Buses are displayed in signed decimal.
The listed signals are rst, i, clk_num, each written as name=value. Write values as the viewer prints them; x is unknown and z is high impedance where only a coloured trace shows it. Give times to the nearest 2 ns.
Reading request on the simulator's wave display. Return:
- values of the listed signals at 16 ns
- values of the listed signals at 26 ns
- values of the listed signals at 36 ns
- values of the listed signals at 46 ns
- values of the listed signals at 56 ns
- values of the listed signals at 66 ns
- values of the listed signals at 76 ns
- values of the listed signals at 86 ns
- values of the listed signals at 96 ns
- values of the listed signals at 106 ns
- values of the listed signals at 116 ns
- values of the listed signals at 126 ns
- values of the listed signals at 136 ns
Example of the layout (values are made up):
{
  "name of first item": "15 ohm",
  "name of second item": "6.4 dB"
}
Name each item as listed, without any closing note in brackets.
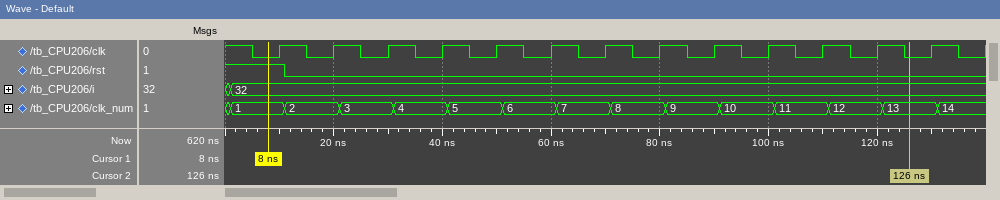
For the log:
{
  "values of the listed signals at 16 ns": "rst=0, i=32, clk_num=2",
  "values of the listed signals at 26 ns": "rst=0, i=32, clk_num=3",
  "values of the listed signals at 36 ns": "rst=0, i=32, clk_num=4",
  "values of the listed signals at 46 ns": "rst=0, i=32, clk_num=5",
  "values of the listed signals at 56 ns": "rst=0, i=32, clk_num=6",
  "values of the listed signals at 66 ns": "rst=0, i=32, clk_num=7",
  "values of the listed signals at 76 ns": "rst=0, i=32, clk_num=8",
  "values of the listed signals at 86 ns": "rst=0, i=32, clk_num=9",
  "values of the listed signals at 96 ns": "rst=0, i=32, clk_num=10",
  "values of the listed signals at 106 ns": "rst=0, i=32, clk_num=11",
  "values of the listed signals at 116 ns": "rst=0, i=32, clk_num=12",
  "values of the listed signals at 126 ns": "rst=0, i=32, clk_num=13",
  "values of the listed signals at 136 ns": "rst=0, i=32, clk_num=14"
}
